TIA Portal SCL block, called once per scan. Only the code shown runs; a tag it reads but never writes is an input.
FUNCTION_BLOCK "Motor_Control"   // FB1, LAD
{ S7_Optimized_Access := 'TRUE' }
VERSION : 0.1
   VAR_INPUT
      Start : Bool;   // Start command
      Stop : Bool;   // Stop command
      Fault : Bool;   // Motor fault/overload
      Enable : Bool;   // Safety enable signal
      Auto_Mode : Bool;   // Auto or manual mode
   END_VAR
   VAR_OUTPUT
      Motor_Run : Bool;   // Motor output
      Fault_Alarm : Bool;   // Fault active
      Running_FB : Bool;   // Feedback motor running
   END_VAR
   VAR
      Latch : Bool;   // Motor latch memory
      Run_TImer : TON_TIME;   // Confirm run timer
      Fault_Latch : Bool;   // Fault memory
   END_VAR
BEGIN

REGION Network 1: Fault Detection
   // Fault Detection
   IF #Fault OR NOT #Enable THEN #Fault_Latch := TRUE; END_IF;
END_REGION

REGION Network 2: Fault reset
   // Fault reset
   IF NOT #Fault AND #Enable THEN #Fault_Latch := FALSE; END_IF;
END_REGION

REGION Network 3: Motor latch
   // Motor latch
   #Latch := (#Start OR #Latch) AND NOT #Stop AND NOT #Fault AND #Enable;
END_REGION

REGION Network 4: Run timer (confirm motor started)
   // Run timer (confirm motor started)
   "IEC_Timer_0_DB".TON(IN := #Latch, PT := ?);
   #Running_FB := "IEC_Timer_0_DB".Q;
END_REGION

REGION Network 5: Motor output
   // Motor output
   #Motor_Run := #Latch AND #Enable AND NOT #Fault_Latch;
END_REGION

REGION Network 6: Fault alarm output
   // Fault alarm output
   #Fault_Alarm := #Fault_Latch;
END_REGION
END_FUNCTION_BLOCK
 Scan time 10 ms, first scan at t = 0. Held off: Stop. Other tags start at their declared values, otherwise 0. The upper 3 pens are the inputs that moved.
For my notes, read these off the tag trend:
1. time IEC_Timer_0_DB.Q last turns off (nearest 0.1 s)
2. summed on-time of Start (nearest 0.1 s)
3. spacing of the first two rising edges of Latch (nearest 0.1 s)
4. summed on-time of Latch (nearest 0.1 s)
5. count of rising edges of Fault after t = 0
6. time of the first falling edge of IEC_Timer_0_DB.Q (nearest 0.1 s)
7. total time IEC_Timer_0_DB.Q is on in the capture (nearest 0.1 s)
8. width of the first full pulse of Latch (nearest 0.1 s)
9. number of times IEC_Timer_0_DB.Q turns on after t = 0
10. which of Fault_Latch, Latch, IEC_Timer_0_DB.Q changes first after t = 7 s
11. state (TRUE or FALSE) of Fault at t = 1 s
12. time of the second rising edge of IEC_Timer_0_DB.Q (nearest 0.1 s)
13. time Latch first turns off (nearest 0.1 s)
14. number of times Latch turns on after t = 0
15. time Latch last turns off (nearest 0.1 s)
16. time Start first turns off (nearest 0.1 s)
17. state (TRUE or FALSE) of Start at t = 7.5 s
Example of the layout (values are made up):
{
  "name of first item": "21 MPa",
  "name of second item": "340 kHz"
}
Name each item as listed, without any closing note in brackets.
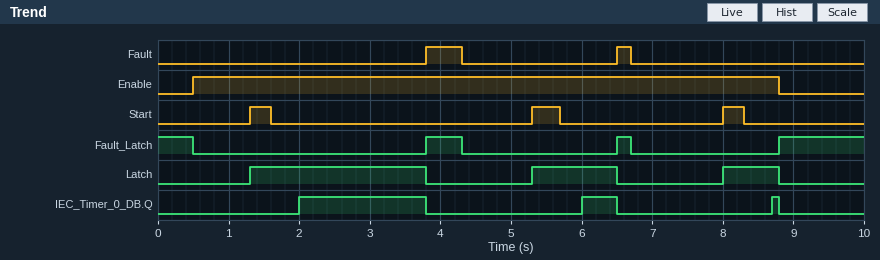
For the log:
{
  "time IEC_Timer_0_DB.Q last turns off": "8.8 s",
  "summed on-time of Start": "1.0 s",
  "spacing of the first two rising edges of Latch": "4.0 s",
  "summed on-time of Latch": "4.5 s",
  "count of rising edges of Fault after t = 0": "2",
  "time of the first falling edge of IEC_Timer_0_DB.Q": "3.8 s",
  "total time IEC_Timer_0_DB.Q is on in the capture": "2.4 s",
  "width of the first full pulse of Latch": "2.5 s",
  "number of times IEC_Timer_0_DB.Q turns on after t = 0": "3",
  "which of Fault_Latch, Latch, IEC_Timer_0_DB.Q changes first after t = 7 s": "Latch",
  "state (TRUE or FALSE) of Fault at t = 1 s": "FALSE",
  "time of the second rising edge of IEC_Timer_0_DB.Q": "6.0 s",
  "time Latch first turns off": "3.8 s",
  "number of times Latch turns on after t = 0": "3",
  "time Latch last turns off": "8.8 s",
  "time Start first turns off": "1.6 s",
  "state (TRUE or FALSE) of Start at t = 7.5 s": "FALSE"
}
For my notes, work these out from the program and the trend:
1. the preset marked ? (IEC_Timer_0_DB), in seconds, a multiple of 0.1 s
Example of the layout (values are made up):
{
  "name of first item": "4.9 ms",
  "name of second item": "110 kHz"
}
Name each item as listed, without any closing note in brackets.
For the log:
{
  "the preset marked ? (IEC_Timer_0_DB), in seconds, a multiple of 0.1 s": "0.7 s"
}
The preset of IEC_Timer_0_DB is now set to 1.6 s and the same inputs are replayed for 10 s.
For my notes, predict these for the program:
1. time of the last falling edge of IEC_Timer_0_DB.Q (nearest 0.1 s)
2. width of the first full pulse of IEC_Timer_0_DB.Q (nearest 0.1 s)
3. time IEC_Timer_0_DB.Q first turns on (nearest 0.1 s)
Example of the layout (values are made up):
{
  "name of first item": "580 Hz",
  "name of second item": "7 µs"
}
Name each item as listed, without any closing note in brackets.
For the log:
{
  "time of the last falling edge of IEC_Timer_0_DB.Q": "3.8 s",
  "width of the first full pulse of IEC_Timer_0_DB.Q": "0.9 s",
  "time IEC_Timer_0_DB.Q first turns on": "2.9 s"
}
